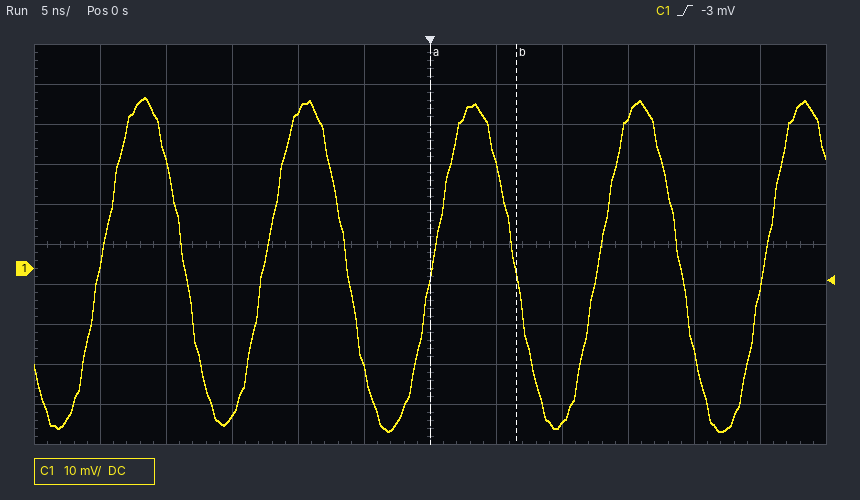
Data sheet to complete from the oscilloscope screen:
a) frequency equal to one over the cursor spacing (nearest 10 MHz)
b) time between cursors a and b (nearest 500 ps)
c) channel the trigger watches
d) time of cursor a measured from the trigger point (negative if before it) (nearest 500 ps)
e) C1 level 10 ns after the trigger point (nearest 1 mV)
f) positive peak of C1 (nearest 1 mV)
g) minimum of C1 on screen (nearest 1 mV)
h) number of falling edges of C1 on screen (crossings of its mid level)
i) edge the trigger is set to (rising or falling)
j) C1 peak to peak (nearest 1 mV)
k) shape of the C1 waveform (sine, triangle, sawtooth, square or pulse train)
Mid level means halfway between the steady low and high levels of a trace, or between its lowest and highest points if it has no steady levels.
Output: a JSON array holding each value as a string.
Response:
["150 MHz", "6.5 ns", "C1", "0.0 ns", "-39 mV", "43 mV", "-41 mV", "4", "rising", "84 mV", "sine"]
